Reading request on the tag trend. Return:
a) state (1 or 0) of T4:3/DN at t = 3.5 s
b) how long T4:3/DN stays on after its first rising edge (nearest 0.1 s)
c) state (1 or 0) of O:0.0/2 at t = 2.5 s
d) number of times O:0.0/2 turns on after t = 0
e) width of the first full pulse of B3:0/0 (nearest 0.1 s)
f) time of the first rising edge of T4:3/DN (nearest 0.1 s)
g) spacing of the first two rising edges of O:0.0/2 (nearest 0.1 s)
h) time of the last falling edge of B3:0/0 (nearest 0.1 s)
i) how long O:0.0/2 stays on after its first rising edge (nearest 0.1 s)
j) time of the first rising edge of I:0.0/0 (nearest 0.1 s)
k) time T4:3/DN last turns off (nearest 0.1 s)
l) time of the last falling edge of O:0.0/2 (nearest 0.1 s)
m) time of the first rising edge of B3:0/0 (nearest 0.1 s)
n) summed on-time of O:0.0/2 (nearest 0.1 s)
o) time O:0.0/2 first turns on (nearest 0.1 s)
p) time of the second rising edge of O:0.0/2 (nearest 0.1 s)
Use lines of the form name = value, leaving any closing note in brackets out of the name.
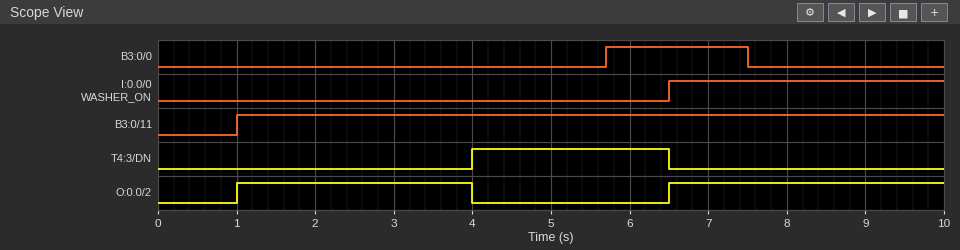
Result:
state (1 or 0) of T4:3/DN at t = 3.5 s = 0
how long T4:3/DN stays on after its first rising edge = 2.5 s
state (1 or 0) of O:0.0/2 at t = 2.5 s = 1
number of times O:0.0/2 turns on after t = 0 = 2
width of the first full pulse of B3:0/0 = 1.8 s
time of the first rising edge of T4:3/DN = 4.0 s
spacing of the first two rising edges of O:0.0/2 = 5.5 s
time of the last falling edge of B3:0/0 = 7.5 s
how long O:0.0/2 stays on after its first rising edge = 3.0 s
time of the first rising edge of I:0.0/0 = 6.5 s
time T4:3/DN last turns off = 6.5 s
time of the last falling edge of O:0.0/2 = 4.0 s
time of the first rising edge of B3:0/0 = 5.7 s
summed on-time of O:0.0/2 = 6.5 s
time O:0.0/2 first turns on = 1.0 s
time of the second rising edge of O:0.0/2 = 6.5 s
